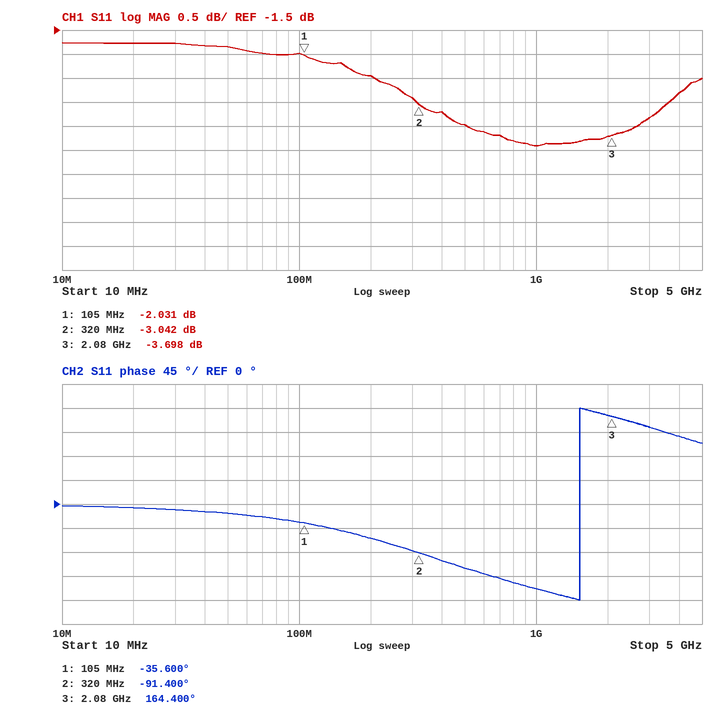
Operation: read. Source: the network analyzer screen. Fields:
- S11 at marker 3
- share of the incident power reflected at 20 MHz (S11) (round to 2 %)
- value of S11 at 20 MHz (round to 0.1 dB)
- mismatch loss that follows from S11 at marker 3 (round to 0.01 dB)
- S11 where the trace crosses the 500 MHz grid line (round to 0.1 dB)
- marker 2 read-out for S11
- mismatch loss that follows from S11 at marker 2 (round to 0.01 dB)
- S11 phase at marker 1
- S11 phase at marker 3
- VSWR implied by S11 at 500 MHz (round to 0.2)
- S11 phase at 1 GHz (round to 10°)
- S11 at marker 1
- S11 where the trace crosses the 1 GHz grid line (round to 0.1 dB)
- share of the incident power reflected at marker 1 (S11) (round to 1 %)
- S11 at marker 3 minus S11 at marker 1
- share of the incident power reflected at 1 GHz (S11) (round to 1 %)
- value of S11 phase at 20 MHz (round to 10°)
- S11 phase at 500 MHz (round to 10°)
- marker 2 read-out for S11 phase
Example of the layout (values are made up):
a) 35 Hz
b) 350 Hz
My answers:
a) -3.698 dB
b) 66 %
c) -1.8 dB
d) 2.42 dB
e) -3.5 dB
f) -3.042 dB
g) 2.98 dB
h) -35.600°
i) 164.400°
j) 5.0
k) -160°
l) -2.031 dB
m) -3.9 dB
n) 63 %
o) -1.667 dB
p) 41 %
q) -10°
r) -120°
s) -91.400°
